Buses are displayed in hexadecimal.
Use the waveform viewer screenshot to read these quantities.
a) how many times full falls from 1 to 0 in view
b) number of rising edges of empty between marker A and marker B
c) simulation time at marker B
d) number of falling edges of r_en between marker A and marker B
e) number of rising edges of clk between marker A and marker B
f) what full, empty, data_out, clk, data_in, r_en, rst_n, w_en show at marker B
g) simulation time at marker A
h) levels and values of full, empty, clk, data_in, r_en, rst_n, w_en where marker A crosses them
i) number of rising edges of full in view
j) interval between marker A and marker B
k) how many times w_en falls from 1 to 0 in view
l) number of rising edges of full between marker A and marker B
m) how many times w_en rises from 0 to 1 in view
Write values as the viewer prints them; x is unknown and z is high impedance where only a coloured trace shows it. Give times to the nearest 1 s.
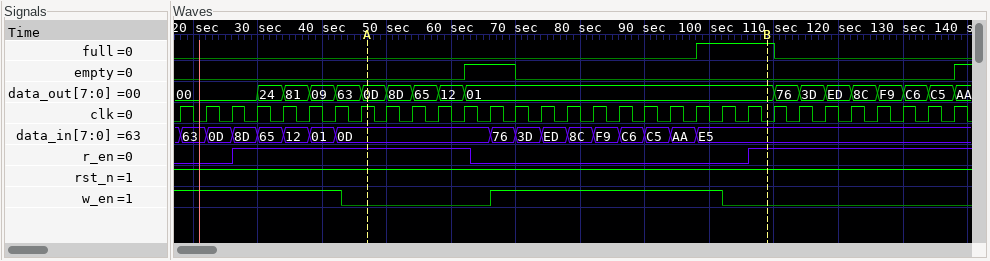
1
1
109 s
1
15
full=1, empty=0, data_out=01, clk=0, data_in=E5, r_en=1, rst_n=1, w_en=0
47 s
full=0, empty=0, clk=1, data_in=0D, r_en=1, rst_n=1, w_en=0
1
62 s
2
1
1
